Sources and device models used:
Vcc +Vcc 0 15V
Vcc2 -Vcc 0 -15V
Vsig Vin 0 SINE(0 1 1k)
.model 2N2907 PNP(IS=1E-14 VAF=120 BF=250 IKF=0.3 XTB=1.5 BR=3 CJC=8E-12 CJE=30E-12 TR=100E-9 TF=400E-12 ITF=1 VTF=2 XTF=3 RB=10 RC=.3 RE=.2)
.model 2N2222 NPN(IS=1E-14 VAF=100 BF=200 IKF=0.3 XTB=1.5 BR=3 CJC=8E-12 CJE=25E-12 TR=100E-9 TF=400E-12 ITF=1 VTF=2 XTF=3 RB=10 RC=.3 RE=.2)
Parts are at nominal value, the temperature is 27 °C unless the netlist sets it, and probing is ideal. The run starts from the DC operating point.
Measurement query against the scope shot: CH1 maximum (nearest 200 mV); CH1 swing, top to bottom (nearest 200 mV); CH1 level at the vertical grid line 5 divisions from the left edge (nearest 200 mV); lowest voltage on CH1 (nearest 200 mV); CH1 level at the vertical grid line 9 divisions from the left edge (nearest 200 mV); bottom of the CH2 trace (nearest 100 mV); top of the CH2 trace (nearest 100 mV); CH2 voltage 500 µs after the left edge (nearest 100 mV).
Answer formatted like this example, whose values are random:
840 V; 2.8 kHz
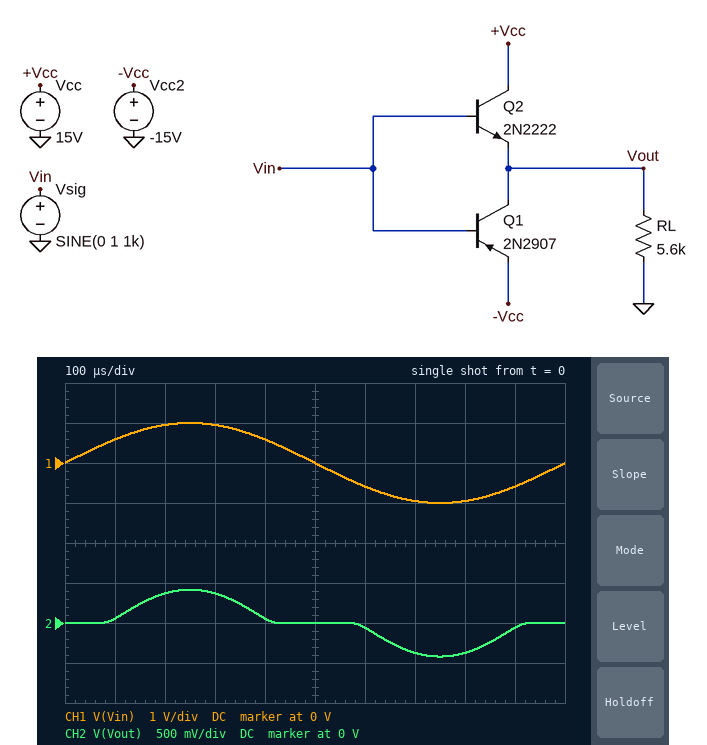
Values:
1.0 V; 2.0 V; 0 V; -1.0 V; -600 mV; -400 mV; 400 mV; 0 V
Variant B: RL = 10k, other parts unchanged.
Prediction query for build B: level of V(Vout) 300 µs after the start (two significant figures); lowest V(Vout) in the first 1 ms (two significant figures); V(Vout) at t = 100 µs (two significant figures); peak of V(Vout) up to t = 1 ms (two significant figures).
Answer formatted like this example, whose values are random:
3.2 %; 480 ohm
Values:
380 mV; -430 mV; 66 mV; 430 mV
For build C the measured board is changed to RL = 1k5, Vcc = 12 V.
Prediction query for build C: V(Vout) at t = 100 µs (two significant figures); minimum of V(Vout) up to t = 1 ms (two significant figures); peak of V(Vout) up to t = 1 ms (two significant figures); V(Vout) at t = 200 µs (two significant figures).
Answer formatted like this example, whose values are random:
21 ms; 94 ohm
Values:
34 mV; -390 mV; 380 mV; 340 mV
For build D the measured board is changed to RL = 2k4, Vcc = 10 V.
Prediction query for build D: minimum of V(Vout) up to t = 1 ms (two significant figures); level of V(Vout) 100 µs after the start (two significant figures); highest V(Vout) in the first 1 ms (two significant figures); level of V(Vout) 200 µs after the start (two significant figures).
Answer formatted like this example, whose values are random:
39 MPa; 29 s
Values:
-400 mV; 41 mV; 390 mV; 350 mV
